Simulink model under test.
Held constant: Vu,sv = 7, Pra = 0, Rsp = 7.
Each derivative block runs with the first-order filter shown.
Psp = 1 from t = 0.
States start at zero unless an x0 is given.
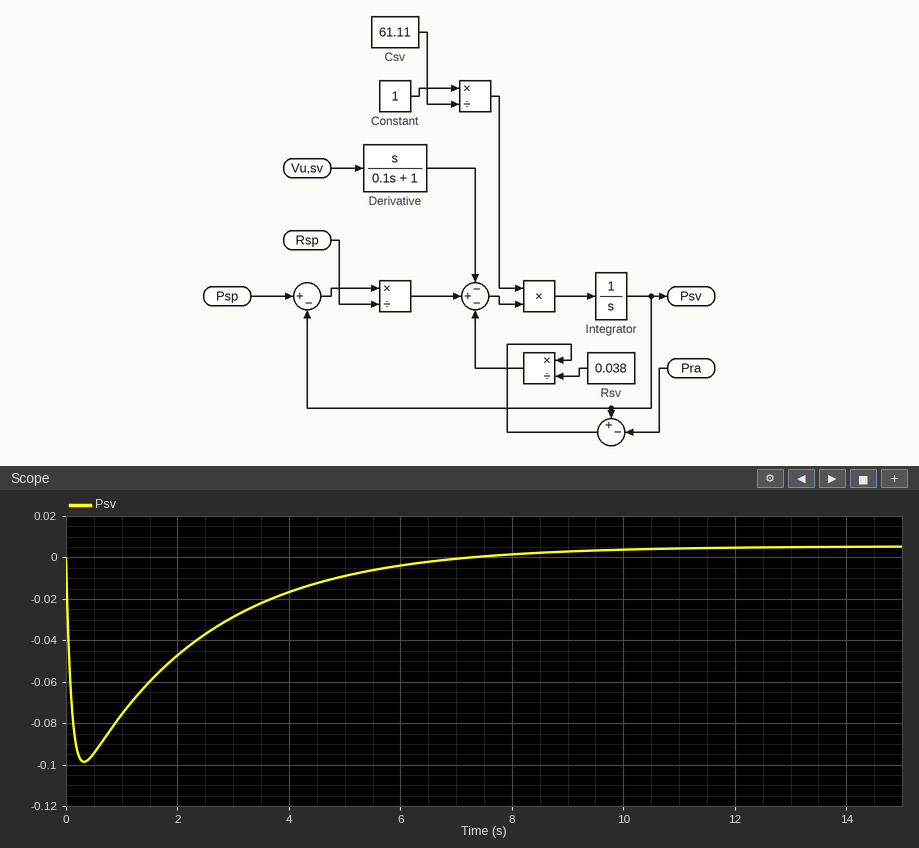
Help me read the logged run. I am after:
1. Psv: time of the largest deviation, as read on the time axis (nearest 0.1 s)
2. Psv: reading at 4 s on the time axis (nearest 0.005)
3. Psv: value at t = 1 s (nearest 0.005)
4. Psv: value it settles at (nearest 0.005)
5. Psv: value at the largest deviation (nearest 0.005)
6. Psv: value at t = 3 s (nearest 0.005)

0.3 s
-0.015
-0.075
0.005
-0.100
-0.030
